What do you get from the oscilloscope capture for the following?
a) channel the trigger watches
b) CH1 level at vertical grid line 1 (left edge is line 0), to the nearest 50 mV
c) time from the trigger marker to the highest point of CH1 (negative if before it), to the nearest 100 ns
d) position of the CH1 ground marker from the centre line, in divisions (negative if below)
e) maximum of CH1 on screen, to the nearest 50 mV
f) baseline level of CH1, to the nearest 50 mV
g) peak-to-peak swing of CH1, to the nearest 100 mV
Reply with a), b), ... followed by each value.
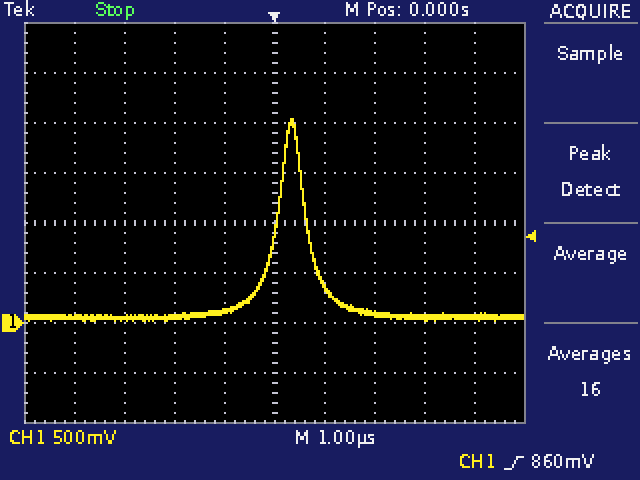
a) CH1
b) 50 mV
c) +300 ns
d) -2.0 div
e) 2.05 V
f) 50 mV
g) 2.00 V
